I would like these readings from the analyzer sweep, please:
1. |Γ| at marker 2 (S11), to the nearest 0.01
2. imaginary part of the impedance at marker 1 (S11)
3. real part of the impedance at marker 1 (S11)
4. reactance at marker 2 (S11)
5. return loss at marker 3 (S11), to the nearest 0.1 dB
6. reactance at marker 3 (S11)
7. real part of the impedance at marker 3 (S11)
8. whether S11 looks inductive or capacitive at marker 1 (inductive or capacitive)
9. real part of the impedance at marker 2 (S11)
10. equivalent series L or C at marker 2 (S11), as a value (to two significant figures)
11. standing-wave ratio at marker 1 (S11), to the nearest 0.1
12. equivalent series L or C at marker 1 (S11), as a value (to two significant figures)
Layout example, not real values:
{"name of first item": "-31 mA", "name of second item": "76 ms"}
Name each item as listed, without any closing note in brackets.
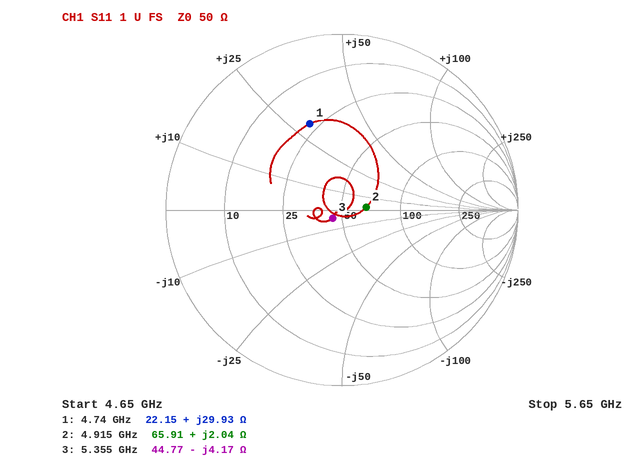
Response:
{"|Γ| at marker 2 (S11), to the nearest 0.01": "0.14", "imaginary part of the impedance at marker 1": "+29.93 Ω", "real part of the impedance at marker 1": "22.15 Ω", "reactance at marker 2": "+2.04 Ω", "return loss at marker 3 (S11), to the nearest 0.1 dB": "23.0 dB", "reactance at marker 3": "-4.17 Ω", "real part of the impedance at marker 3": "44.77 Ω", "whether S11 looks inductive or capacitive at marker 1": "inductive", "real part of the impedance at marker 2": "65.91 Ω", "equivalent series L or C at marker 2 (S11), as a value": "66 pH", "standing-wave ratio at marker 1 (S11), to the nearest 0.1": "3.2", "equivalent series L or C at marker 1 (S11), as a value": "1.0 nH"}
